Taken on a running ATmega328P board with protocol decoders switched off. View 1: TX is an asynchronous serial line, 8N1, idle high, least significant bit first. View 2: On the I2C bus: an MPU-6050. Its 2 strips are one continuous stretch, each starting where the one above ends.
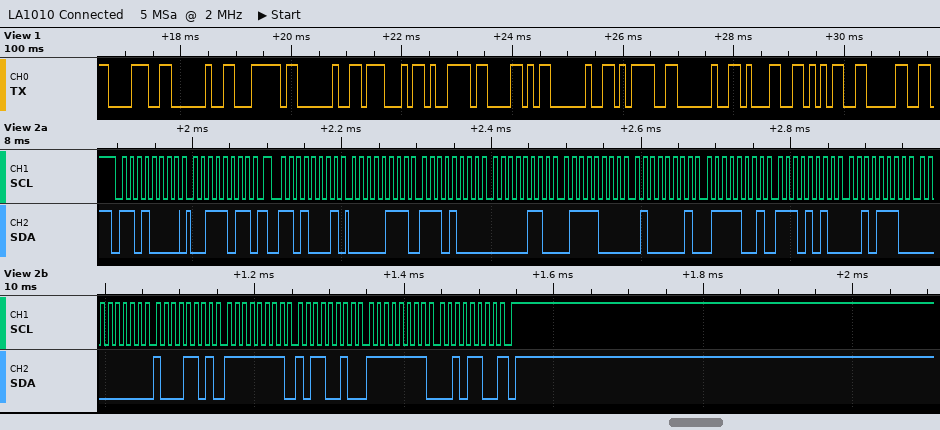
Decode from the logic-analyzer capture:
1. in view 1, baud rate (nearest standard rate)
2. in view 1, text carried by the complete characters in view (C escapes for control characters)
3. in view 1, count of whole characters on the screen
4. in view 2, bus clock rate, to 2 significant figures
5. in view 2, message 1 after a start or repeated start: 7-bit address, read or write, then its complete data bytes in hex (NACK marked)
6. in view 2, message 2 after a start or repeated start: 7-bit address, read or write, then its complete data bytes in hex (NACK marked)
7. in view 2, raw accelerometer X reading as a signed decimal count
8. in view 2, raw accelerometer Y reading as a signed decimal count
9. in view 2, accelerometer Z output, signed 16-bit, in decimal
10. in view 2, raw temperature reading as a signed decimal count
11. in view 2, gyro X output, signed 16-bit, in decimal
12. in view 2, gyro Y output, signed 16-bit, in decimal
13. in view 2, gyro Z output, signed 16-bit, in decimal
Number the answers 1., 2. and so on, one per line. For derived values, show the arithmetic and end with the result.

1. 9600 baud
2. "8 | GyX = 150"
3. 13
4. 100 kHz
5. 0x68 write: 3B
6. 0x68 read: 07 E8 06 78 41 79 EA 2E 00 8D FF B2 FF 2C NACK
7. 0x07E8 = 2024
8. 0x0678 = 1656
9. 0x4179 = 16761
10. 0xEA2E = -5586
11. 0x008D = 141
12. 0xFFB2 = -78
13. 0xFF2C = -212
